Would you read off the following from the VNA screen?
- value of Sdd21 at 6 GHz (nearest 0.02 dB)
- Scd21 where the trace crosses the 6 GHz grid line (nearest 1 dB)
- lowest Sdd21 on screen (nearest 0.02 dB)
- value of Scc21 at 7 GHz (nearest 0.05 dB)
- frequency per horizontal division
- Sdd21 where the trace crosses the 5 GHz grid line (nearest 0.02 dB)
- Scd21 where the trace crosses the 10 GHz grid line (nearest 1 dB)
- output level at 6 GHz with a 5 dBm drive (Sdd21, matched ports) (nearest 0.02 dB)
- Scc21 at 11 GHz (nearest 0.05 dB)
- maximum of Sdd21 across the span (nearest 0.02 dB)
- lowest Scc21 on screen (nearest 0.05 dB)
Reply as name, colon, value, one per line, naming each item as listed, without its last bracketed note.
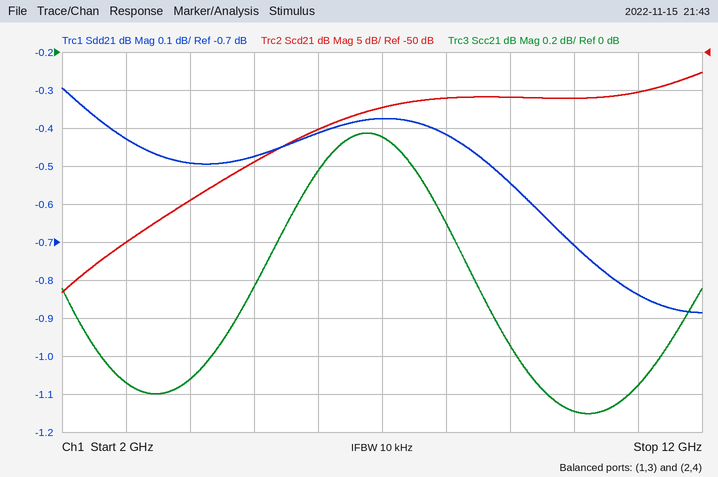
value of Sdd21 at 6 GHz: -0.42 dB
Scd21 where the trace crosses the 6 GHz grid line: -60 dB
lowest Sdd21 on screen: -0.88 dB
value of Scc21 at 7 GHz: -0.45 dB
frequency per horizontal division: 1 GHz
Sdd21 where the trace crosses the 5 GHz grid line: -0.48 dB
Scd21 where the trace crosses the 10 GHz grid line: -56 dB
output level at 6 GHz with a 5 dBm drive (Sdd21, matched ports): 4.58 dBm
Scc21 at 11 GHz: -1.75 dB
maximum of Sdd21 across the span: -0.30 dB
lowest Scc21 on screen: -1.90 dB
